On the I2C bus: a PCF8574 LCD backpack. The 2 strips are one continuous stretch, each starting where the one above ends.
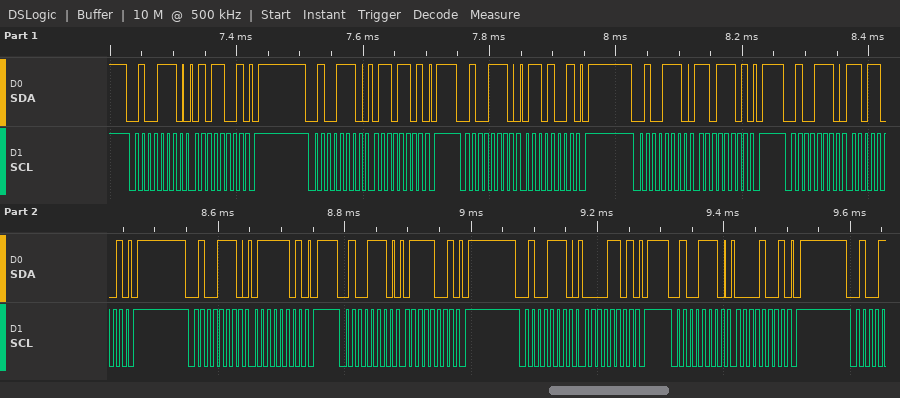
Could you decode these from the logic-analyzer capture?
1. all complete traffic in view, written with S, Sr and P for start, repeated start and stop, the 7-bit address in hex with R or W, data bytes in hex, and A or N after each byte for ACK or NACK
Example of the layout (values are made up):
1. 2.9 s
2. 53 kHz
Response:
1. S 27W A 59 A P S 27W A 6D A P S 27W A 69 A P S 27W A DD A P S 27W A D9 A P S 27W A 7D A P S 27W A 79 A P S 27W A 0D A P S 27W A 09 A P
